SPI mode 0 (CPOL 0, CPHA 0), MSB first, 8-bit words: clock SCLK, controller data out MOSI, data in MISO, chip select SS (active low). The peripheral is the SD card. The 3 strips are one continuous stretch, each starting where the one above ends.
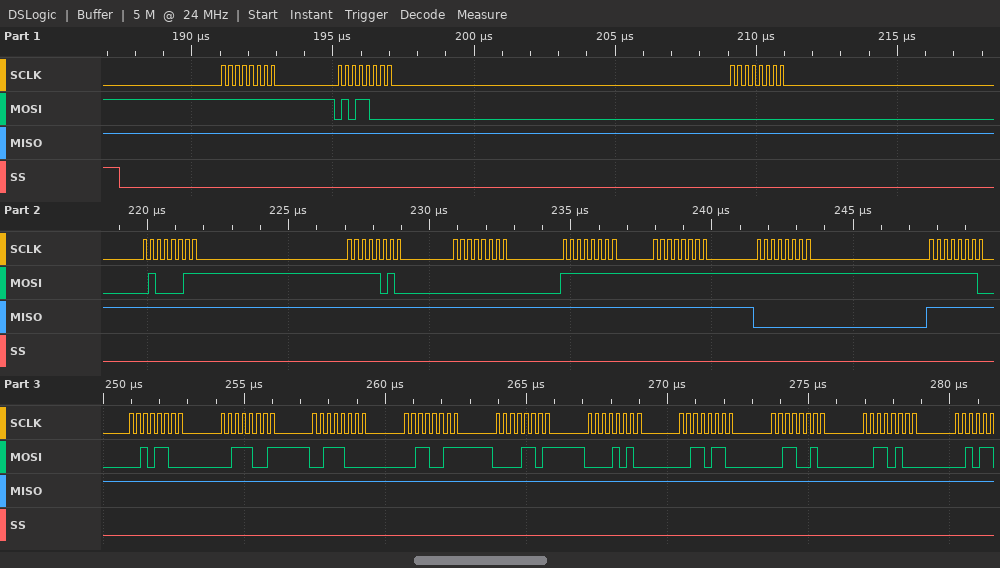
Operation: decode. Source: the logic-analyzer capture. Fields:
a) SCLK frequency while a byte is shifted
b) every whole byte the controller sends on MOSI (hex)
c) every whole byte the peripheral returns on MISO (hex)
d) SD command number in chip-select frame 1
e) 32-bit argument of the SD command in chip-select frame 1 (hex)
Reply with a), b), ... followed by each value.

a) 4 MHz
b) 0xFF 0x58 0x00 0x43 0xFA 0x00 0xFF 0xFF 0xFF 0xFE 0x2C 0x39 0x38 0x33 0x0D 0x0A 0x36 0x32 0x34
c) 0xFF 0xFF 0xFF 0xFF 0xFF 0xFF 0xFF 0xFF 0x00 0xFF 0xFF 0xFF 0xFF 0xFF 0xFF 0xFF 0xFF 0xFF 0xFF
d) CMD24
e) 0x0043FA00
